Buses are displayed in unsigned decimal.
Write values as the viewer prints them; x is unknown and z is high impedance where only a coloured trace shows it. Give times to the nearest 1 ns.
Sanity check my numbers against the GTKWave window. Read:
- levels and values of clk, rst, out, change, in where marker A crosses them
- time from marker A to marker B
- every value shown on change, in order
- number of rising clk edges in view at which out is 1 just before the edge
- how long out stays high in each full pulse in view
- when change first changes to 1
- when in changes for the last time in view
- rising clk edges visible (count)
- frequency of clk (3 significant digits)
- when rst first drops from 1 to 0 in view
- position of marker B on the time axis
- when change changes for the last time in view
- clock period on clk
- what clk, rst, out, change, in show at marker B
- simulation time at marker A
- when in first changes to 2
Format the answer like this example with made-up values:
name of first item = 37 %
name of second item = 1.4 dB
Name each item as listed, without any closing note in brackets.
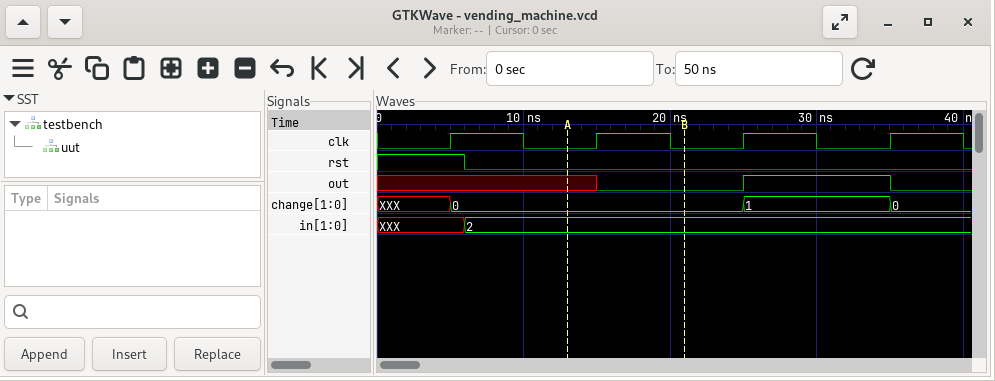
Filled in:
levels and values of clk, rst, out, change, in where marker A crosses them = clk=0, rst=0, out=x, change=0, in=2
time from marker A to marker B = 8 ns
every value shown on change, in order = XXX, 0, 1, 0
number of rising clk edges in view at which out is 1 just before the edge = 1
how long out stays high in each full pulse in view = 10 ns
when change first changes to 1 = 25 ns
when in changes for the last time in view = 6 ns
rising clk edges visible = 4
frequency of clk = 100 MHz
when rst first drops from 1 to 0 in view = 6 ns
position of marker B on the time axis = 21 ns
when change changes for the last time in view = 35 ns
clock period on clk = 10 ns
what clk, rst, out, change, in show at marker B = clk=0, rst=0, out=0, change=0, in=2
simulation time at marker A = 13 ns
when in first changes to 2 = 6 ns
